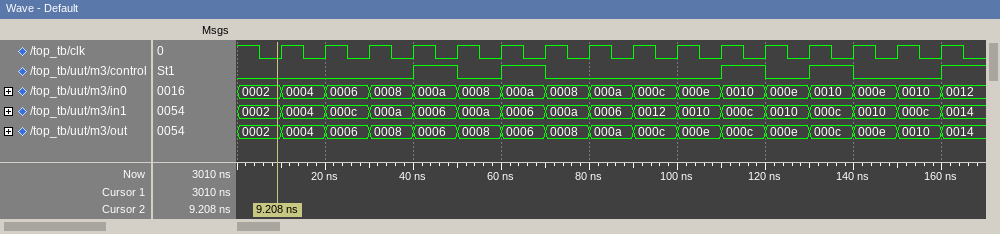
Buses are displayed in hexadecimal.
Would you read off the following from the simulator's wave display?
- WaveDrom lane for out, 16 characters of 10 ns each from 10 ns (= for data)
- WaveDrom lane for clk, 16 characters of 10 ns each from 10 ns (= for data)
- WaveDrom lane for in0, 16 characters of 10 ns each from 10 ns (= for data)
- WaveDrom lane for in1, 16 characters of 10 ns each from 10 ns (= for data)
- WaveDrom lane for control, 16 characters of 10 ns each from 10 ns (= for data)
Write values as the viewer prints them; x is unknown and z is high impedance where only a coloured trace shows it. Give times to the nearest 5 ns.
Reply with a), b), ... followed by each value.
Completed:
a) {name: 'out', wave: '================', data: '0004 0006 0008 0006 0008 0006 0008 000a 000c 000e 000c 000e 000c 000e 0010 0014'}
b) {name: 'clk', wave: 'p...............'}
c) {name: 'in0', wave: '================', data: '0004 0006 0008 000a 0008 000a 0008 000a 000c 000e 0010 000e 0010 000e 0010 0012'}
d) {name: 'in1', wave: '================', data: '0004 000c 000a 0006 000a 0006 000a 0006 0012 0010 000c 0010 000c 0010 000c 0014'}
e) {name: 'control', wave: '0..1010...1010.1'}
